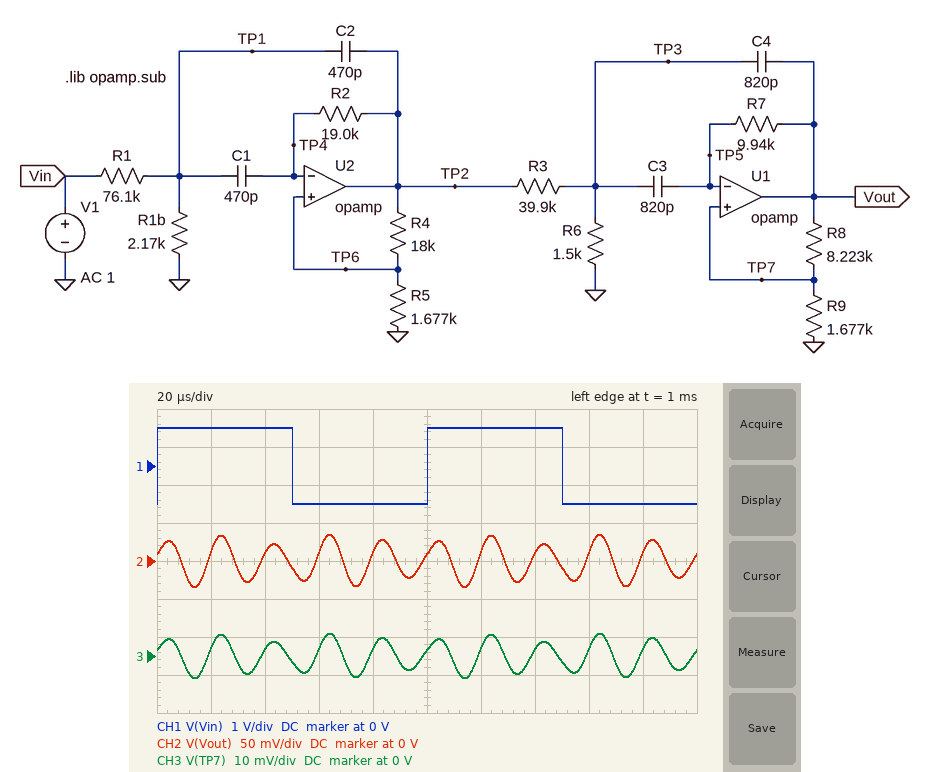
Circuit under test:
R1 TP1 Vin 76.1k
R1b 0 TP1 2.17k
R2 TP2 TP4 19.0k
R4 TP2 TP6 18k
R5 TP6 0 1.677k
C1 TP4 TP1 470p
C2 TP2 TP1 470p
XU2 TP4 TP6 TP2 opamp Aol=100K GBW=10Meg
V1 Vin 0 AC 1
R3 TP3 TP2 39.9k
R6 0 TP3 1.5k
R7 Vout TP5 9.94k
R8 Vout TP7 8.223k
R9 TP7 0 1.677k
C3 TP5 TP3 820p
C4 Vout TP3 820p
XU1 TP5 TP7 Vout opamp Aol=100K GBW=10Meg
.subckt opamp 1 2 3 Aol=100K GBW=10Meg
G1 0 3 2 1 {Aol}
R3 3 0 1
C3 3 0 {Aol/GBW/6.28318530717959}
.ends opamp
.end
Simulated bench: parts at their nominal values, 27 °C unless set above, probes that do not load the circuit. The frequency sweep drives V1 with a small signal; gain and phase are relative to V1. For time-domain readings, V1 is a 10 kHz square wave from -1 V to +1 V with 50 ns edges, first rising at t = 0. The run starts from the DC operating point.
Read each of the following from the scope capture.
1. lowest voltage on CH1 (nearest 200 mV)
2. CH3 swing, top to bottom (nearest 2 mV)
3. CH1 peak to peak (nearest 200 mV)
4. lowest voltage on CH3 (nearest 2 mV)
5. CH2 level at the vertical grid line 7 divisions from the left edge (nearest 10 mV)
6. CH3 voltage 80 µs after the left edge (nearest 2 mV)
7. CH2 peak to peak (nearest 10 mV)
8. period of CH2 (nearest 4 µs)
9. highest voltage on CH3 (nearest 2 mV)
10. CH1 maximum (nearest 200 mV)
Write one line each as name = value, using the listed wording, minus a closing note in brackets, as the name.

lowest voltage on CH1 = -1.0 V
CH3 swing, top to bottom = 12 mV
CH1 peak to peak = 2.0 V
lowest voltage on CH3 = -6 mV
CH2 level at the vertical grid line 7 divisions from the left edge = 10 mV
CH3 voltage 80 µs after the left edge = 2 mV
CH2 peak to peak = 70 mV
period of CH2 = 20 µs
highest voltage on CH3 = 6 mV
CH1 maximum = 1.0 V
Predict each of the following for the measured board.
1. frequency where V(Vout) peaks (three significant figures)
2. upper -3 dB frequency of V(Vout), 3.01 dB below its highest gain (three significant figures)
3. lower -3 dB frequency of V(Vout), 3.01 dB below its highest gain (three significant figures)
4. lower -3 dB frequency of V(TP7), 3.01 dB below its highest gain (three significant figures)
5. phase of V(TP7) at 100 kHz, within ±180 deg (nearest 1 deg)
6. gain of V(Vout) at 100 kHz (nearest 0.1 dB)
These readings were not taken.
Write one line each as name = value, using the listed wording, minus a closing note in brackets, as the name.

frequency where V(Vout) peaks = 51.3 kHz
upper -3 dB frequency of V(Vout), 3.01 dB below its highest gain = 56.4 kHz
lower -3 dB frequency of V(Vout), 3.01 dB below its highest gain = 46.9 kHz
lower -3 dB frequency of V(TP7), 3.01 dB below its highest gain = 46.9 kHz
phase of V(TP7) at 100 kHz, within ±180 deg = -157 deg
gain of V(Vout) at 100 kHz = -46.2 dB
